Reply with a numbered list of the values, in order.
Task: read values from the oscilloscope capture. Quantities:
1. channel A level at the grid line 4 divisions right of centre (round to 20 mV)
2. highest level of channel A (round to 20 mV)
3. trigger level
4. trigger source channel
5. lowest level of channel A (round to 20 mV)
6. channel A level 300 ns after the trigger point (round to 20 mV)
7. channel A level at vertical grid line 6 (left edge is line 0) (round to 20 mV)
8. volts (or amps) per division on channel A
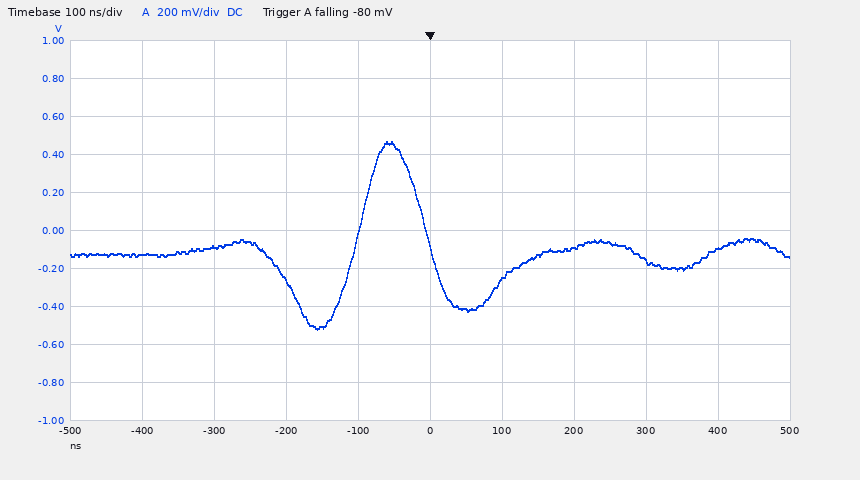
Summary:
1. -100 mV
2. 460 mV
3. -80 mV
4. channel A
5. -520 mV
6. -160 mV
7. -260 mV
8. 200 mV
